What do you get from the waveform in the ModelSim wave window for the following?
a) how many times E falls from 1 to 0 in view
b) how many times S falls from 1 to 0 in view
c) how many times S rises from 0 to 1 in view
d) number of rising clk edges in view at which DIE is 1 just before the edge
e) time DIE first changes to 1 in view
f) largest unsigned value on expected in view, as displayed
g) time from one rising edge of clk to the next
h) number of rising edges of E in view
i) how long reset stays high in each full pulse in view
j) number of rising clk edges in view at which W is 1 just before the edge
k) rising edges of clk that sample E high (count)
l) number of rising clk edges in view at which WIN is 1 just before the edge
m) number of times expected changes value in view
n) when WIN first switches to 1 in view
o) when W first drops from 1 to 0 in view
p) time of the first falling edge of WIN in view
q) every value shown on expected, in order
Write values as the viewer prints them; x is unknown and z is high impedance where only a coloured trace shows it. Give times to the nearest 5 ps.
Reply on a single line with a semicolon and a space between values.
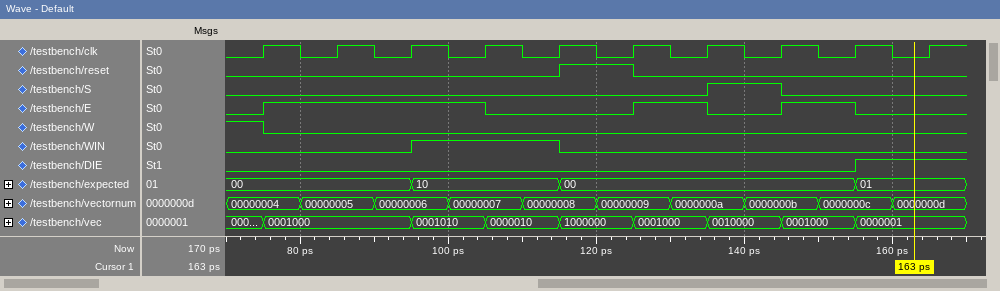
3; 1; 1; 1; 155 ps; 10; 10 ps; 3; 10 ps; 1; 5; 2; 3; 95 ps; 75 ps; 115 ps; 00, 10, 00, 01
